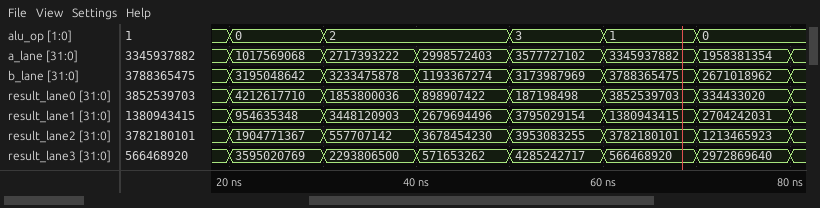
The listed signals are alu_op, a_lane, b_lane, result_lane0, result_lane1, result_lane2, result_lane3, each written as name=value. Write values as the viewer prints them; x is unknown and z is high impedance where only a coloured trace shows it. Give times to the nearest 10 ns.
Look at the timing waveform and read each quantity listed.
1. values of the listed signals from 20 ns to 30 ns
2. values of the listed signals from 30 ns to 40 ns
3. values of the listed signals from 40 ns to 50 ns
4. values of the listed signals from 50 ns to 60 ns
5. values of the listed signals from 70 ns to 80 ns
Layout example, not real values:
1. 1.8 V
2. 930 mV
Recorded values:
1. alu_op=0, a_lane=1017569068, b_lane=3195048642, result_lane0=4212617710, result_lane1=954635348, result_lane2=1904771367, result_lane3=3595020769
2. alu_op=2, a_lane=2717393222, b_lane=3233475878, result_lane0=1853800036, result_lane1=3448120903, result_lane2=557707142, result_lane3=2293806500
3. alu_op=2, a_lane=2998572403, b_lane=1193367274, result_lane0=898907422, result_lane1=2679694496, result_lane2=3678454230, result_lane3=571653262
4. alu_op=3, a_lane=3577727102, b_lane=3173987969, result_lane0=187198498, result_lane1=3795029154, result_lane2=3953083255, result_lane3=4285242717
5. alu_op=0, a_lane=1958381354, b_lane=2671018962, result_lane0=334433020, result_lane1=2704242031, result_lane2=1213465923, result_lane3=2972869640
